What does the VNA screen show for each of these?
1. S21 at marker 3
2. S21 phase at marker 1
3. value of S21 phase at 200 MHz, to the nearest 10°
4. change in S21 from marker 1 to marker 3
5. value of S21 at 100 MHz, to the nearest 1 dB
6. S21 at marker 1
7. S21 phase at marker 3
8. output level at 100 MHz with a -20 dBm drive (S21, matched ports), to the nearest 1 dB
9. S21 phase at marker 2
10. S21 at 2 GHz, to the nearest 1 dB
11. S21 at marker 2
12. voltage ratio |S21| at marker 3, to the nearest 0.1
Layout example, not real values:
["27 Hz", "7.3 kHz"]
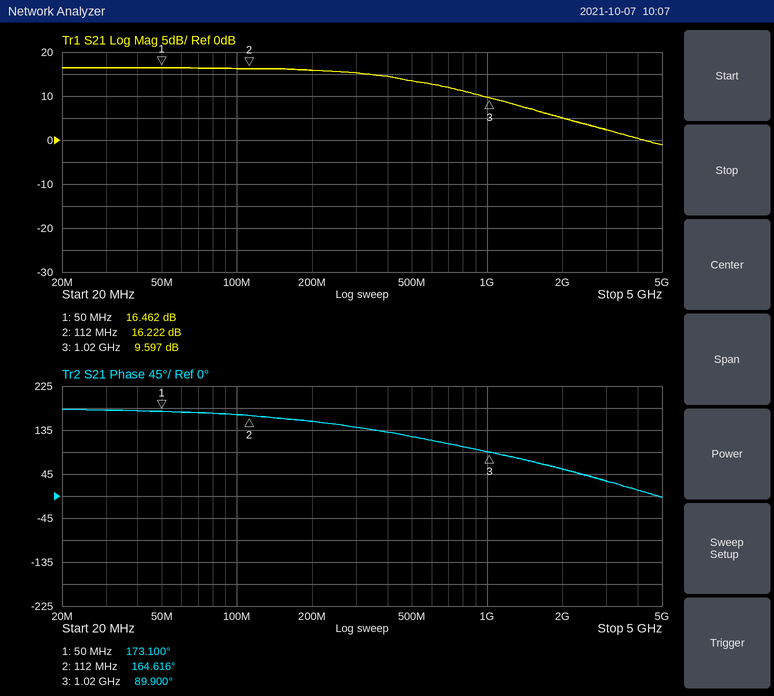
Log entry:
["9.597 dB", "173.100°", "150°", "-6.865 dB", "16 dB", "16.462 dB", "89.900°", "-4 dBm", "164.616°", "5 dB", "16.222 dB", "3.0"]
